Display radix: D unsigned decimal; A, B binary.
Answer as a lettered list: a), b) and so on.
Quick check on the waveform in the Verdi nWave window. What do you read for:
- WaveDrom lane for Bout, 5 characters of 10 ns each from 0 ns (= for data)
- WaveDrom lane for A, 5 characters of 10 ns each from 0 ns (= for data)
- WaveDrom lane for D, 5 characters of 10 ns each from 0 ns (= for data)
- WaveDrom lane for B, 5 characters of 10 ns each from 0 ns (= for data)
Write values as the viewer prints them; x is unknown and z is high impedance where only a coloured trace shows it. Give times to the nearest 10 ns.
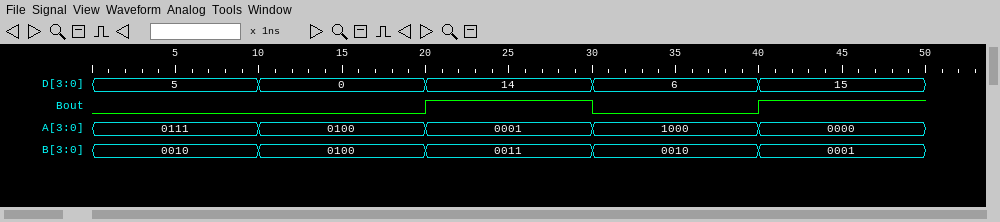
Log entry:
a) {name: 'Bout', wave: '0.101'}
b) {name: 'A', wave: '=====', data: '0111 0100 0001 1000 0000'}
c) {name: 'D', wave: '=====', data: '5 0 14 6 15'}
d) {name: 'B', wave: '=====', data: '0010 0100 0011 0010 0001'}
